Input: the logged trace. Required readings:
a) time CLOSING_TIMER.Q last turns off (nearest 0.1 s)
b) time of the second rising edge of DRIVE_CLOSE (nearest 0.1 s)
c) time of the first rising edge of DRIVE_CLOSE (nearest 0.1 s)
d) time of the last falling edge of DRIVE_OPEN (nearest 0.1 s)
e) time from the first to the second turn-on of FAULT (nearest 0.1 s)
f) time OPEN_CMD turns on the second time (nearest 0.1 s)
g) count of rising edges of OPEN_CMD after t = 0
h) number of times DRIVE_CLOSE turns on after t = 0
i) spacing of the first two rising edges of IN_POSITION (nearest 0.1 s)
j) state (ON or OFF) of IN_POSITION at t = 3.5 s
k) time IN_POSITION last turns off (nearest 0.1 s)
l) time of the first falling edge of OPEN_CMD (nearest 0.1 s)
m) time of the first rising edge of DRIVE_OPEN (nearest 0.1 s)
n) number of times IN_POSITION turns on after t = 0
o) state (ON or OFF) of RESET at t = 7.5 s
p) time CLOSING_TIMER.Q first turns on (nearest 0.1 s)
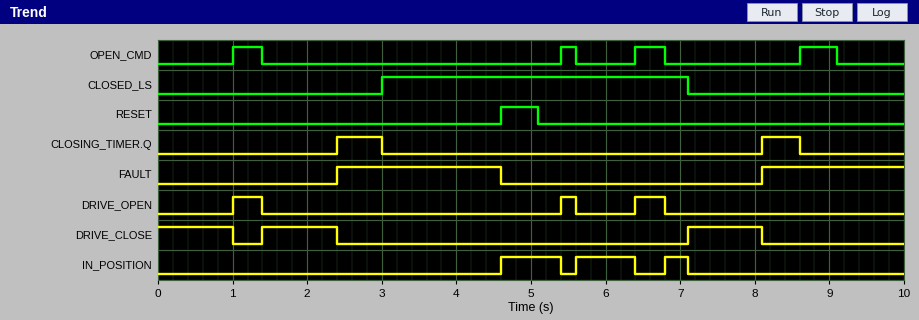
8.6 s
7.1 s
1.4 s
6.8 s
5.7 s
5.4 s
4
2
1.0 s
OFF
7.1 s
1.4 s
1.0 s
3
OFF
2.4 s
